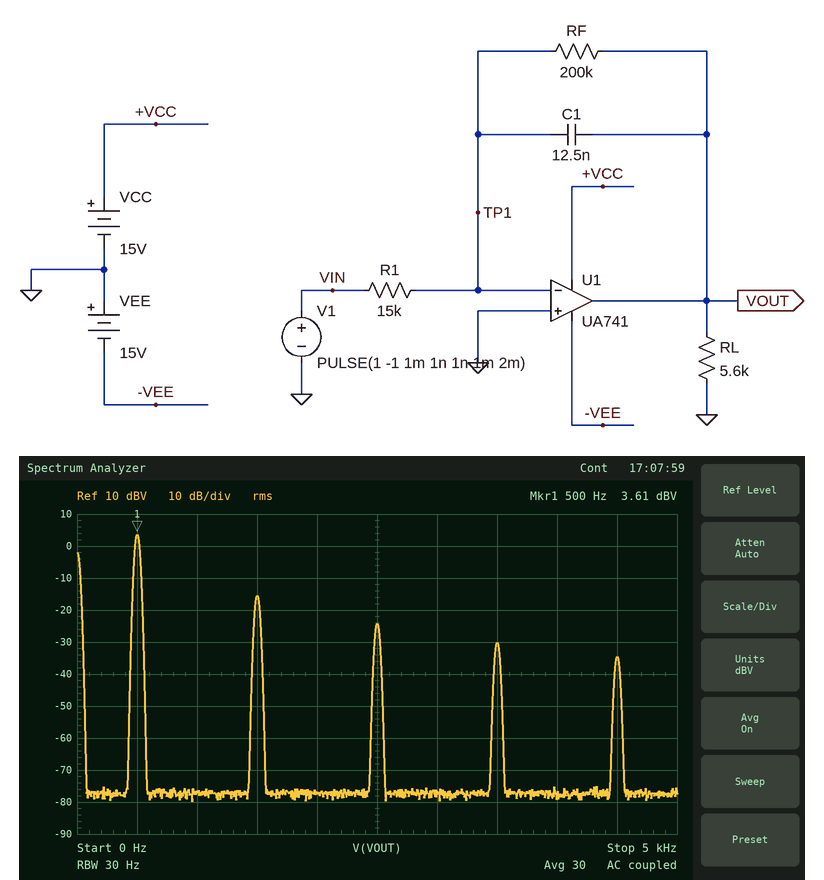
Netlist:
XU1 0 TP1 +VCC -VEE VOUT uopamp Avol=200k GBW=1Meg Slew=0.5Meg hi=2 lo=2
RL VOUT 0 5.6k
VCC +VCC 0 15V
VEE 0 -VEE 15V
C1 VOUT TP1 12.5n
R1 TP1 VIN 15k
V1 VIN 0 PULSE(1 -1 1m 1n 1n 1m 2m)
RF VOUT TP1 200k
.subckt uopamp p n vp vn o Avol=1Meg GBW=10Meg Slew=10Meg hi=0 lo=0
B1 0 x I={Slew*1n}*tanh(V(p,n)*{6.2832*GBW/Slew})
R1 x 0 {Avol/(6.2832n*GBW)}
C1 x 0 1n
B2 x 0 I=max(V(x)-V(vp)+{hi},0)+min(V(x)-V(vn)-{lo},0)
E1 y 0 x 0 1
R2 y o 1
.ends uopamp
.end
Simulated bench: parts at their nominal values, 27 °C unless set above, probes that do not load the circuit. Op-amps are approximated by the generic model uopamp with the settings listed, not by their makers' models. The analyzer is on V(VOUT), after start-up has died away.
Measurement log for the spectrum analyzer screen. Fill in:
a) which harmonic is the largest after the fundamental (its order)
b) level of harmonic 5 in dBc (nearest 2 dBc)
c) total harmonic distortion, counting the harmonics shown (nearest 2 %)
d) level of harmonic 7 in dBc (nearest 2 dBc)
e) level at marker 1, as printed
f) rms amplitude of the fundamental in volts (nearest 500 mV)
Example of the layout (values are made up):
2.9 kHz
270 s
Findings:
3
-28 dBc
12 %
-34 dBc
3.61 dBV
1.5 V
